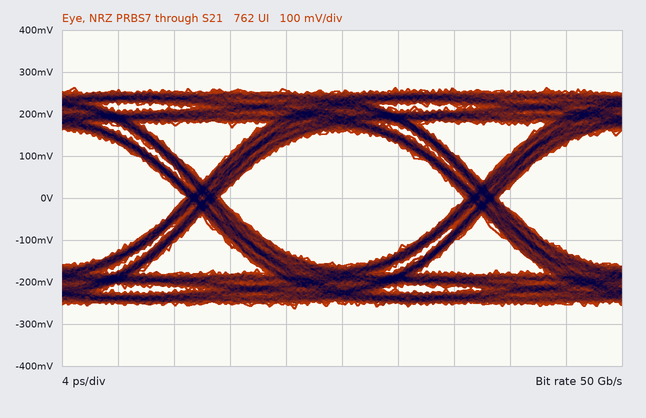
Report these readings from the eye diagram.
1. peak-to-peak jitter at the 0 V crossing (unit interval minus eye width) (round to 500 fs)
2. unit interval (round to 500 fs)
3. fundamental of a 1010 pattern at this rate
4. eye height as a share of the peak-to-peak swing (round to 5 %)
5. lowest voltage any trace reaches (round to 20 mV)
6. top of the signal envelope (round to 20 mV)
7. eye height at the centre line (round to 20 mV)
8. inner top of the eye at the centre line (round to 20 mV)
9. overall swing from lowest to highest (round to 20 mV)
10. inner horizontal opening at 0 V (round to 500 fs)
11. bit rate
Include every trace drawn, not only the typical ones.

2.5 ps
20.0 ps
25 GHz
60 %
-260 mV
260 mV
320 mV
160 mV
520 mV
17.5 ps
50 Gb/s
